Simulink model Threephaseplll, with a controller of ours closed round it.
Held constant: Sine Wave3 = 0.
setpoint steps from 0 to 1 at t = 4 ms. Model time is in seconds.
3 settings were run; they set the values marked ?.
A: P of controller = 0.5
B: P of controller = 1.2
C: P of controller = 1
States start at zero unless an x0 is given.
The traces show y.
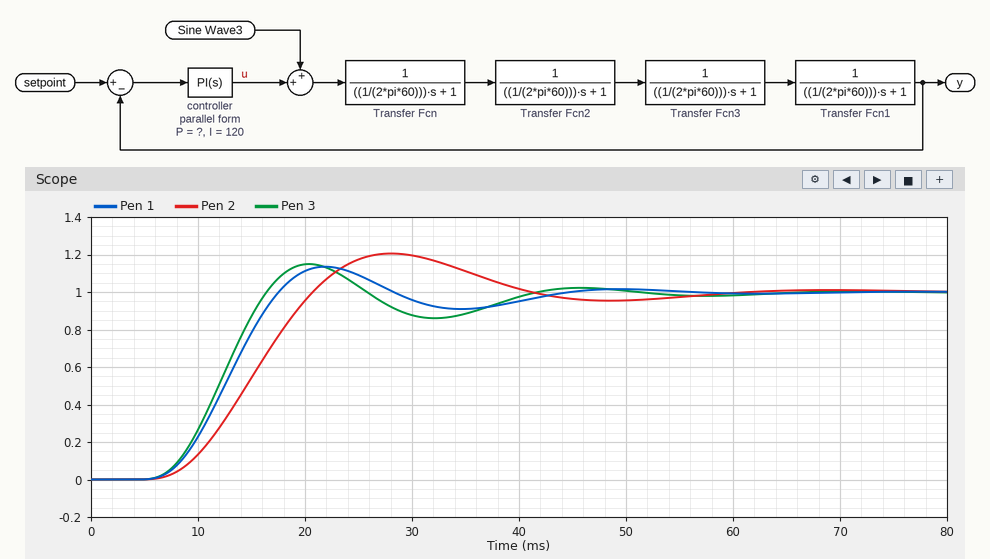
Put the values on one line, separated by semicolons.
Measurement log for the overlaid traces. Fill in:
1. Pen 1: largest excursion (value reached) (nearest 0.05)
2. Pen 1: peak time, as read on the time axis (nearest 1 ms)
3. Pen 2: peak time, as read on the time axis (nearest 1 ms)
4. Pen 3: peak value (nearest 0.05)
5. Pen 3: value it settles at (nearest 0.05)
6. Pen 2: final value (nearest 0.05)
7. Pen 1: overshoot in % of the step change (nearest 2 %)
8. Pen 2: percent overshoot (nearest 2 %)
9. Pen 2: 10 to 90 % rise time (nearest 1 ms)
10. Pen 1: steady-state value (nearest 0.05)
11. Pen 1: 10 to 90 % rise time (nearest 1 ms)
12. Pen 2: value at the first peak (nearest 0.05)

1.15; 22 ms; 28 ms; 1.15; 1.00; 1.00; 14 %; 20 %; 10 ms; 1.00; 8 ms; 1.20
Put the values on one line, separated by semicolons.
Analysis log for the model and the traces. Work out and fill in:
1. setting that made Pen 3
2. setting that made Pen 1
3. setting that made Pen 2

B; C; A
